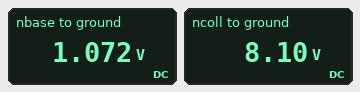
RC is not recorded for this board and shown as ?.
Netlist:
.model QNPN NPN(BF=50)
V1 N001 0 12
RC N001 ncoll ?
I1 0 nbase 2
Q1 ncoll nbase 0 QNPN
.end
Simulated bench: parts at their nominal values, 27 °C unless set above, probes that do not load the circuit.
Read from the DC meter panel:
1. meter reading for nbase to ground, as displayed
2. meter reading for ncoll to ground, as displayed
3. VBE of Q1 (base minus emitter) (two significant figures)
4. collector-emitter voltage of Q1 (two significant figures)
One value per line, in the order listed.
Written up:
1.072 V
8.10 V
1.1 V
8.1 V
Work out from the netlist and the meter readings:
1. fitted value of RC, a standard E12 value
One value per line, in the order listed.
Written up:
0.039 Ω
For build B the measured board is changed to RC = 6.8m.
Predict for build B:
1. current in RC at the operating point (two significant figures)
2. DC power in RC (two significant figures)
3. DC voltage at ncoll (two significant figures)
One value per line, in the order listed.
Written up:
100 A
68 W
11 V
